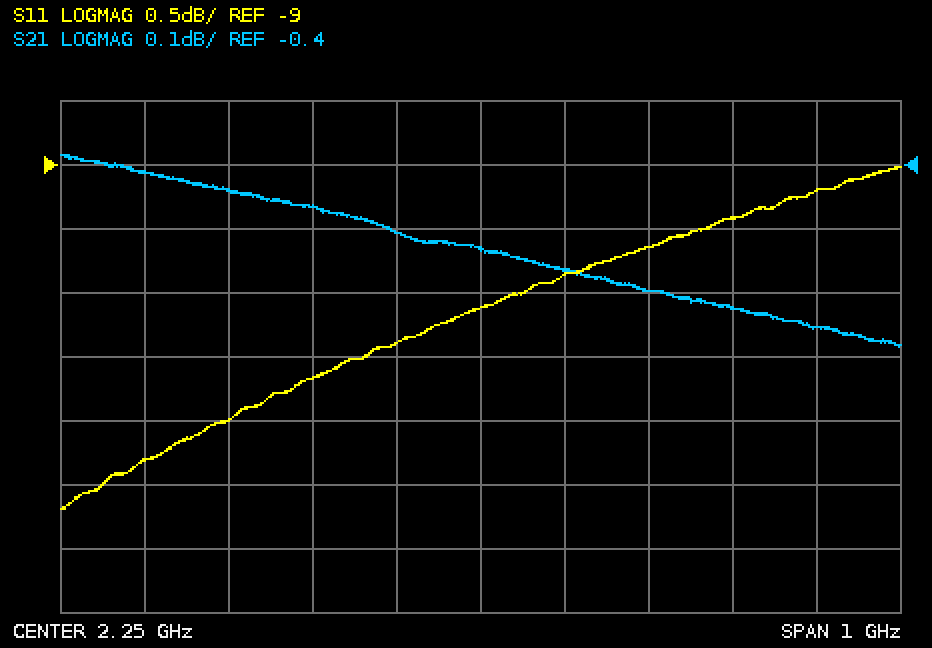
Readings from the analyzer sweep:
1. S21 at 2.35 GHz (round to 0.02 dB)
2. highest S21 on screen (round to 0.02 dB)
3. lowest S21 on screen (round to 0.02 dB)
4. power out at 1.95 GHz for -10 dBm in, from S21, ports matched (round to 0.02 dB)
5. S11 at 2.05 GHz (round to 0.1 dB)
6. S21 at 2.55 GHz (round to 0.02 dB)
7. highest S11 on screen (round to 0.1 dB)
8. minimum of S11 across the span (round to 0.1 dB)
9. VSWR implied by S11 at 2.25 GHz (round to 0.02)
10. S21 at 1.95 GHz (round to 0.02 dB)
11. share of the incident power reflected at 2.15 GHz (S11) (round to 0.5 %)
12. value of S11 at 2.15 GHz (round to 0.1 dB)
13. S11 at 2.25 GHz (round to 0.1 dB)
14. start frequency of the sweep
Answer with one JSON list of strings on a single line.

["-0.56 dB", "-0.38 dB", "-0.68 dB", "-10.44 dBm", "-10.7 dB", "-0.62 dB", "-9.0 dB", "-11.7 dB", "1.90", "-0.44 dB", "9.0 %", "-10.4 dB", "-10.1 dB", "1.75 GHz"]
